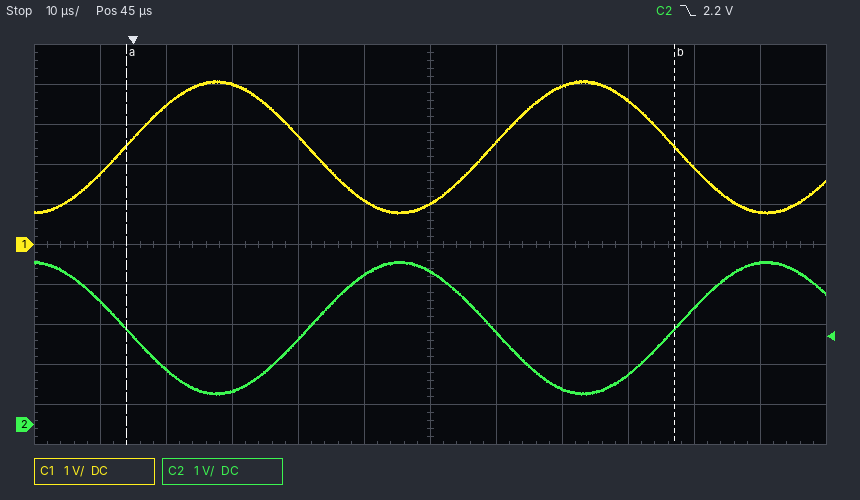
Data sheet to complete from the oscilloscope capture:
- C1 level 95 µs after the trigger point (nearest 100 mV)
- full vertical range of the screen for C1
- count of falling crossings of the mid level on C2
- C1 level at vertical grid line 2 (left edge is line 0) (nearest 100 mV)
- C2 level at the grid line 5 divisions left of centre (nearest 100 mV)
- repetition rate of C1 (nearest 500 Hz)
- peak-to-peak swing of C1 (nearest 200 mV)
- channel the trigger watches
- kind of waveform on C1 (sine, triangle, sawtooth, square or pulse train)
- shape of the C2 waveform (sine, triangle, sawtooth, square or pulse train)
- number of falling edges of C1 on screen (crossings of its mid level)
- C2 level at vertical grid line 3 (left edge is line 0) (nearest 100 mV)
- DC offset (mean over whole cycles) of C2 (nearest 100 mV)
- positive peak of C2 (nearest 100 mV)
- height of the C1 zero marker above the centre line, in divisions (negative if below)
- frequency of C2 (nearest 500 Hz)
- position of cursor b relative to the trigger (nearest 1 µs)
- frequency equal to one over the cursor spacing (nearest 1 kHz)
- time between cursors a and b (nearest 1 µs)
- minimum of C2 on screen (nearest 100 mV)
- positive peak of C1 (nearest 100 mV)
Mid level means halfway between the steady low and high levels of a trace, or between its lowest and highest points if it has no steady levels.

800 mV
10 V
2
3.5 V
3.1 V
18.0 kHz
3.4 V
C2
sine
sine
2
800 mV
2.4 V
4.1 V
0.0 div
18.0 kHz
+82 µs
12 kHz
83 µs
700 mV
4.1 V
